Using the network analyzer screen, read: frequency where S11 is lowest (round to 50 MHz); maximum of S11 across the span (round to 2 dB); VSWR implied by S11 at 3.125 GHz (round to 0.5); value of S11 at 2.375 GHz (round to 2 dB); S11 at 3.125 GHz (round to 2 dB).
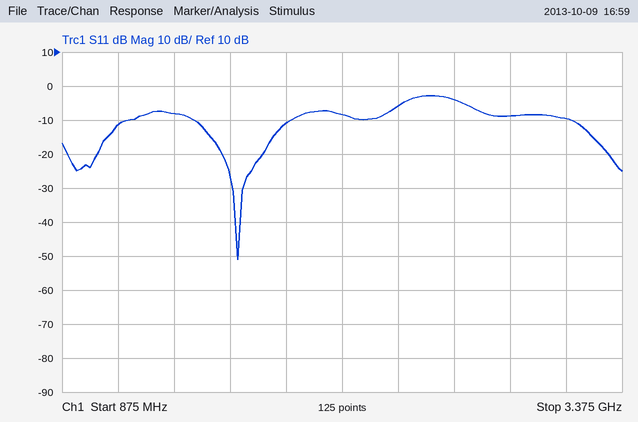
1.65 GHz
-2 dB
2.0
-6 dB
-10 dB
